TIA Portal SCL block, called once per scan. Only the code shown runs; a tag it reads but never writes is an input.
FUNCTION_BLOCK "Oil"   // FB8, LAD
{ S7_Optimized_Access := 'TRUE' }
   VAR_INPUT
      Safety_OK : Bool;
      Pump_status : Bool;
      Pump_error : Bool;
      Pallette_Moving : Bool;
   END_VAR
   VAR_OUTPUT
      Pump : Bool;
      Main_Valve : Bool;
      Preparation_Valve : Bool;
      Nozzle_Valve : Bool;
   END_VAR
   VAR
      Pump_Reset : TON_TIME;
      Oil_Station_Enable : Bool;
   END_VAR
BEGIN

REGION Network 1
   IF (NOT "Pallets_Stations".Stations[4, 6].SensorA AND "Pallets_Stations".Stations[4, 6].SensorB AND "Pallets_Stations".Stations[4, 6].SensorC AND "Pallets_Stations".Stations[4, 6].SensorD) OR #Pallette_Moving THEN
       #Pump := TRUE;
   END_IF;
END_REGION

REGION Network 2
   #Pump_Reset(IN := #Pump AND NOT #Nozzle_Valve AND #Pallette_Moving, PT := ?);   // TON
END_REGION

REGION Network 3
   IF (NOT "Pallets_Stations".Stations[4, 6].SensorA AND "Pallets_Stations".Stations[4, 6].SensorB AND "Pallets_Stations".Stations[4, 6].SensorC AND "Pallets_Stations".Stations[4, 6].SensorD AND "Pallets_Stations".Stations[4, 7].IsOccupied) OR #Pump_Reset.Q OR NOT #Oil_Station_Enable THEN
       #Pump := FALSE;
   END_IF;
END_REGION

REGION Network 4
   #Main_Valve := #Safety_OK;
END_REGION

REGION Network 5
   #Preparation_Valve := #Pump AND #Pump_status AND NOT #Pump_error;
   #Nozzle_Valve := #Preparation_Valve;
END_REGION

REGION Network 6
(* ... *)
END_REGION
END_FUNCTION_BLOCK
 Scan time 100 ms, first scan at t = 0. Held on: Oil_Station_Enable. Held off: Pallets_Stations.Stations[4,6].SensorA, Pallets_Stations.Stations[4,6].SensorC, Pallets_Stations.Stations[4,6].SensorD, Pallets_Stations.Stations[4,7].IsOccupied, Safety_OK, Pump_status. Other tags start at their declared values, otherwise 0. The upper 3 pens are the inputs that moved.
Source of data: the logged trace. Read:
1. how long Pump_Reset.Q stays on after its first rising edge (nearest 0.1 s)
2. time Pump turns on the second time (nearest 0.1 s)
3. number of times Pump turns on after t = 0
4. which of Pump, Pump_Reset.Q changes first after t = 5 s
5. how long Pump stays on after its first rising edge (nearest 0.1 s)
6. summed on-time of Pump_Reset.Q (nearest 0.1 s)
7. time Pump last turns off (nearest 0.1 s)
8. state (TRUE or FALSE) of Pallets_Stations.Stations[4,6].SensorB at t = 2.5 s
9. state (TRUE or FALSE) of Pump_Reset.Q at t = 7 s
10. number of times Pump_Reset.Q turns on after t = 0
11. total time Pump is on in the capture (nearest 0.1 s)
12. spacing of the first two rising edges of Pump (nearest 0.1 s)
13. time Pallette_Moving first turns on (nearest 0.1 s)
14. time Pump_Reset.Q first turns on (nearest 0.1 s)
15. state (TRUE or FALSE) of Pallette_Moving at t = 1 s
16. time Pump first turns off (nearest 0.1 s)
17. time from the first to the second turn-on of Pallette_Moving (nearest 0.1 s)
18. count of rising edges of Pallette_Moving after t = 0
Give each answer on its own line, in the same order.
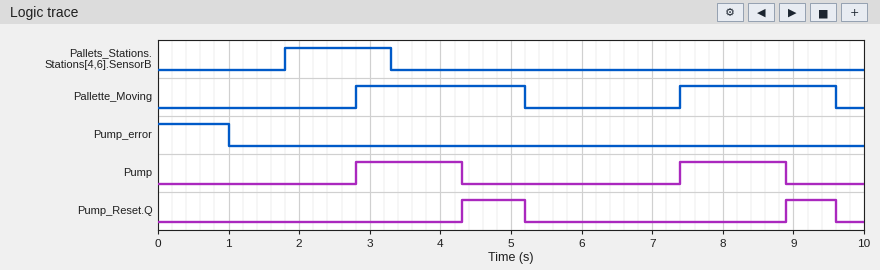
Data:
0.9 s
7.4 s
2
Pump_Reset.Q
1.5 s
1.6 s
8.9 s
TRUE
FALSE
2
3.0 s
4.6 s
2.8 s
4.3 s
FALSE
4.3 s
4.6 s
2
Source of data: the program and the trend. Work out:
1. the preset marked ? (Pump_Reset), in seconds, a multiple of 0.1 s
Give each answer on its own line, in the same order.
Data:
1.5 s
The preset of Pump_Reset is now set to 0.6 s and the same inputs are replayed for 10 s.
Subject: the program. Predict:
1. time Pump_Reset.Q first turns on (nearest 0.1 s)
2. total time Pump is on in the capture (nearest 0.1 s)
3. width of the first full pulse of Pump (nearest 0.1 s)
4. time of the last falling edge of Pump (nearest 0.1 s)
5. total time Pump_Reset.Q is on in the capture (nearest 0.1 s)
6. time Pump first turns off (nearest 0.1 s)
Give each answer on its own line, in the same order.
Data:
3.4 s
1.2 s
0.6 s
8.0 s
3.4 s
3.4 s
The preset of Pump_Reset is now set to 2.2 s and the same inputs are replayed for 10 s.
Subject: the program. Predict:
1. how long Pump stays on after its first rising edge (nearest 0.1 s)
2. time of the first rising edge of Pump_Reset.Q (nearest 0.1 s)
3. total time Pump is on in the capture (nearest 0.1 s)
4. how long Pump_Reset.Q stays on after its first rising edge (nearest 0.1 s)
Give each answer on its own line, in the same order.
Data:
2.2 s
5.0 s
4.8 s
0.2 s
